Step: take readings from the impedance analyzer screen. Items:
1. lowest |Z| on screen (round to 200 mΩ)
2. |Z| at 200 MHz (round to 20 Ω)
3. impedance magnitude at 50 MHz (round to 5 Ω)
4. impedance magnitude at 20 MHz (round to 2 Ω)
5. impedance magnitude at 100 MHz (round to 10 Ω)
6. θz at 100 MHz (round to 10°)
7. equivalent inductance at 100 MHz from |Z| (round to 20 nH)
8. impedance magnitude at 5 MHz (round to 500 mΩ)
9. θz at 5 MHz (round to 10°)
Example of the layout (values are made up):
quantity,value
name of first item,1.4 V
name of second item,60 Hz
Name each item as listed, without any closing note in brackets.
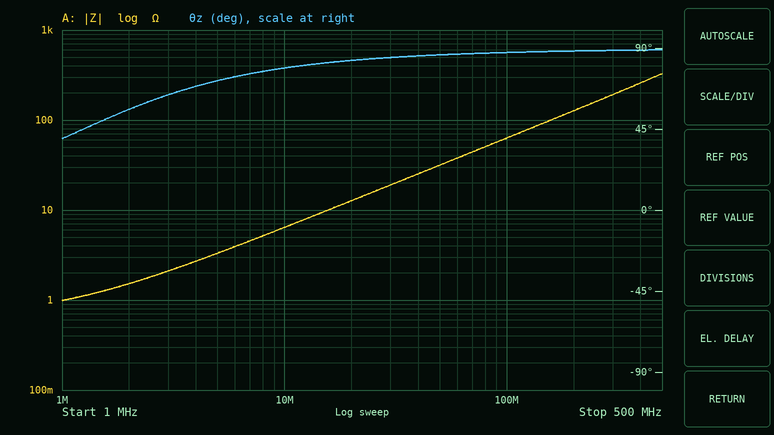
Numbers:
quantity,value
lowest |Z| on screen,1.0 Ω
|Z| at 200 MHz,120 Ω
impedance magnitude at 50 MHz,30 Ω
impedance magnitude at 20 MHz,12 Ω
impedance magnitude at 100 MHz,60 Ω
θz at 100 MHz,90°
equivalent inductance at 100 MHz from |Z|,100 nH
impedance magnitude at 5 MHz,3.5 Ω
θz at 5 MHz,70°
